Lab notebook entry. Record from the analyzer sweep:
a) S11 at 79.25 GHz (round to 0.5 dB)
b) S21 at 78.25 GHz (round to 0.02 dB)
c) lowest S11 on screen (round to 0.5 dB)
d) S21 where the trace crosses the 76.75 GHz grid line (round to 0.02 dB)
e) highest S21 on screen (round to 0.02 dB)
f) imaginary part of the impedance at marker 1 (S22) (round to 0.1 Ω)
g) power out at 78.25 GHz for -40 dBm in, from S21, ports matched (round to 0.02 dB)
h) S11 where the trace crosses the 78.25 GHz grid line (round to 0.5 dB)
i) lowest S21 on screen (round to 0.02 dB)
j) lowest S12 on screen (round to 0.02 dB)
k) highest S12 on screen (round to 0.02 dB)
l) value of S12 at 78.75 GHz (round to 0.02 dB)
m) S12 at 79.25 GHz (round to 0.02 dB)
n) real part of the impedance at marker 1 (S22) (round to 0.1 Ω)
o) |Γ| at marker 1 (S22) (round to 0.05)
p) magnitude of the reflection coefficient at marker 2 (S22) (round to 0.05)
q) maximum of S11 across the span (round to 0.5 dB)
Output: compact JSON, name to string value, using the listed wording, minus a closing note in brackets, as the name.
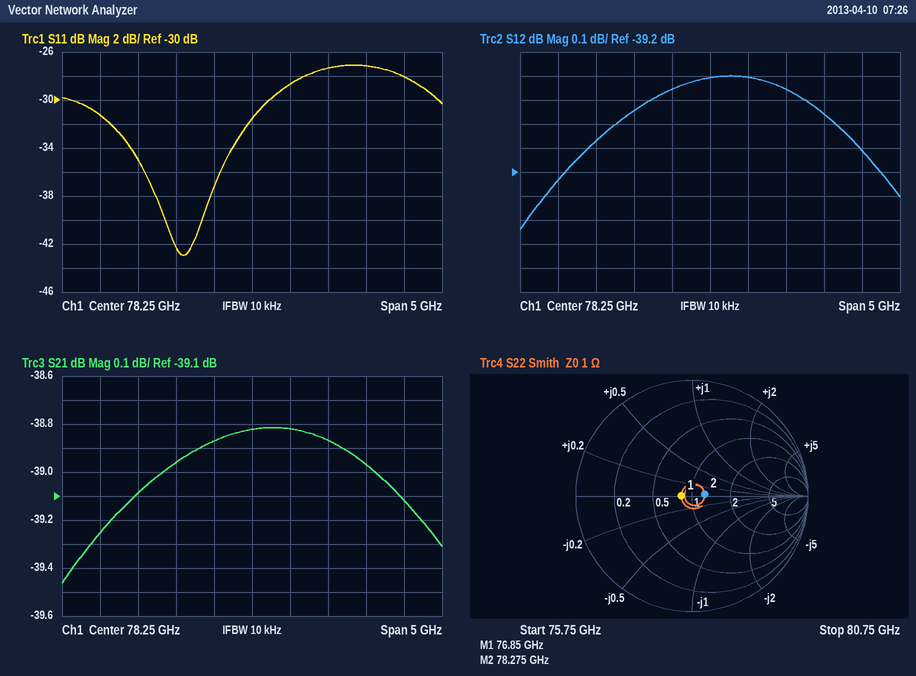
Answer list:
{"S11 at 79.25 GHz": "-27.5 dB", "S21 at 78.25 GHz": "-38.82 dB", "lowest S11 on screen": "-43.0 dB", "S21 where the trace crosses the 76.75 GHz grid line": "-39.08 dB", "highest S21 on screen": "-38.82 dB", "imaginary part of the impedance at marker 1 (S22)": "0.0 Ω", "power out at 78.25 GHz for -40 dBm in, from S21, ports matched": "-78.82 dBm", "S11 where the trace crosses the 78.25 GHz grid line": "-31.5 dB", "lowest S21 on screen": "-39.46 dB", "lowest S12 on screen": "-39.44 dB", "highest S12 on screen": "-38.80 dB", "value of S12 at 78.75 GHz": "-38.80 dB", "S12 at 79.25 GHz": "-38.86 dB", "real part of the impedance at marker 1 (S22)": "0.8 Ω", "|Γ| at marker 1 (S22)": "0.10", "magnitude of the reflection coefficient at marker 2 (S22)": "0.10", "maximum of S11 across the span": "-27.0 dB"}
